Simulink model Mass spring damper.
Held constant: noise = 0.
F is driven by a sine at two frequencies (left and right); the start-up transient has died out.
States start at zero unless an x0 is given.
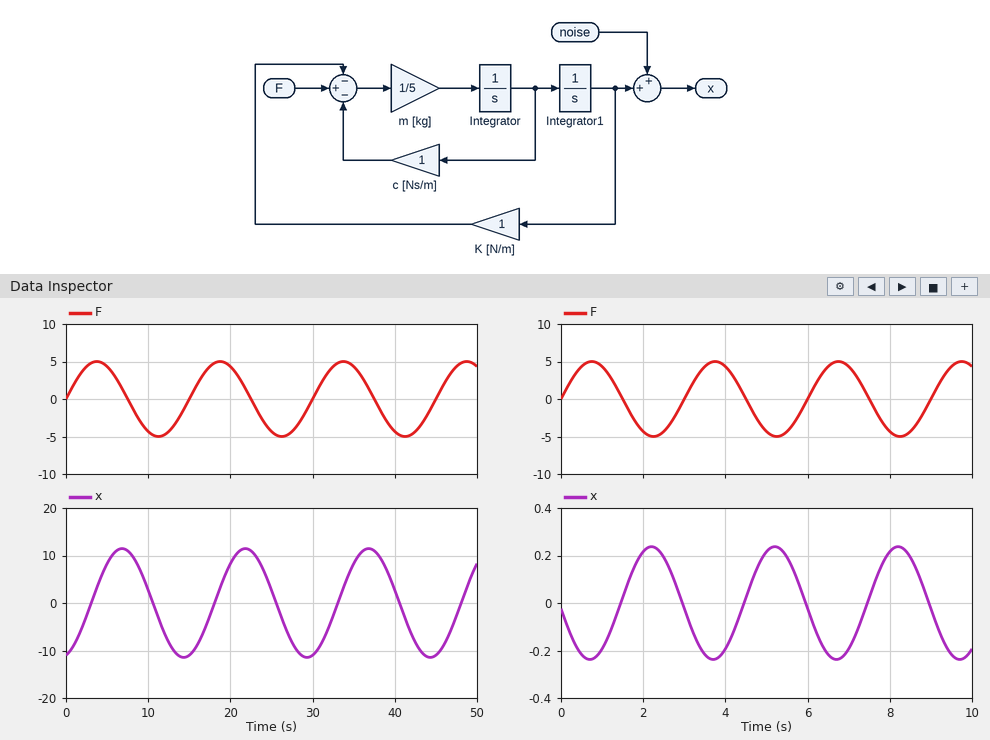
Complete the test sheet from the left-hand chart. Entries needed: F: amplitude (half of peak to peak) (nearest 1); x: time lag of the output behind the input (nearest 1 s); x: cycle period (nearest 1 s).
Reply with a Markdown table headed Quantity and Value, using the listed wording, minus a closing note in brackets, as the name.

| Quantity | Value |
|---|---|
| F: amplitude (half of peak to peak) | 5 |
| x: time lag of the output behind the input | 3 s |
| x: cycle period | 15 s |
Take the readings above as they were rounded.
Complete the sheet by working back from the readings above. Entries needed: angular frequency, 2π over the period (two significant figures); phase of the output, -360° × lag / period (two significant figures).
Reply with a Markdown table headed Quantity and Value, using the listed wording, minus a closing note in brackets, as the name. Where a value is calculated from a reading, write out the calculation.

| Quantity | Value |
|---|---|
| angular frequency, 2π over the period | 2π / 15 = 0.42 rad/s |
| phase of the output, -360° × lag / period | -360 × 3 / 15 = -72° |
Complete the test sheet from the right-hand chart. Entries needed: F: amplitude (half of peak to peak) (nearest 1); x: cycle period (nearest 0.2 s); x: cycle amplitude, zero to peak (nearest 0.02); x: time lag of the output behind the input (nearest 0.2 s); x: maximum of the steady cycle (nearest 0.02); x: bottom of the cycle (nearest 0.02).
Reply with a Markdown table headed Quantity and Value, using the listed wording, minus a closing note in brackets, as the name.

| Quantity | Value |
|---|---|
| F: amplitude (half of peak to peak) | 5 |
| x: cycle period | 3.0 s |
| x: cycle amplitude, zero to peak | 0.24 |
| x: time lag of the output behind the input | 1.4 s |
| x: maximum of the steady cycle | 0.24 |
| x: bottom of the cycle | -0.24 |
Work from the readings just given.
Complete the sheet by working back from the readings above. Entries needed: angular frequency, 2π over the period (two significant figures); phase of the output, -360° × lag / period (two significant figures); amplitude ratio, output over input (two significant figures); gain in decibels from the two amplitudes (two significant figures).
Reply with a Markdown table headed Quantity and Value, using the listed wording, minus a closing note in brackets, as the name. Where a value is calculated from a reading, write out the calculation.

| Quantity | Value |
|---|---|
| angular frequency, 2π over the period | 2π / 3 = 2.1 rad/s |
| phase of the output, -360° × lag / period | -360 × 1.4 / 3 = -170° |
| amplitude ratio, output over input | 0.24 / 5 = 0.048 |
| gain in decibels from the two amplitudes | 20 log10(0.24 / 5) = -26 dB |
